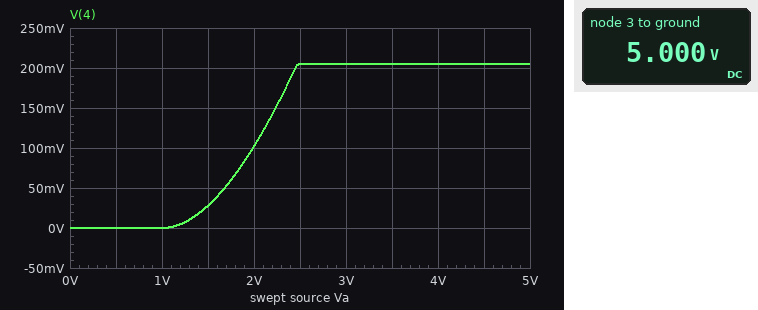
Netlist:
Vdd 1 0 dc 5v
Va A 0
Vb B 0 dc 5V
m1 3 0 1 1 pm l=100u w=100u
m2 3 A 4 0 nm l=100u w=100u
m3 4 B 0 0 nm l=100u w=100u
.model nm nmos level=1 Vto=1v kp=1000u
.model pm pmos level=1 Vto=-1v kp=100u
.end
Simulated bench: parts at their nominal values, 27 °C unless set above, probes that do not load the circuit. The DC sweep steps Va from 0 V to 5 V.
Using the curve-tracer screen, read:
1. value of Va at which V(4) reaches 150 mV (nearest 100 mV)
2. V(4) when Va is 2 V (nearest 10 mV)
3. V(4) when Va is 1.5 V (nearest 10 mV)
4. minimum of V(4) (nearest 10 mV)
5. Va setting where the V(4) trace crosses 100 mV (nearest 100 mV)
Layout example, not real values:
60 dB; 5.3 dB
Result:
2.2 V; 100 mV; 30 mV; 0 V; 2.0 V
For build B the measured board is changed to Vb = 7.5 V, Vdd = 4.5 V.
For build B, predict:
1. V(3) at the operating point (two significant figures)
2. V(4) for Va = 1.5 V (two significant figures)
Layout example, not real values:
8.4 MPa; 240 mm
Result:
4.5 V; 18 mV
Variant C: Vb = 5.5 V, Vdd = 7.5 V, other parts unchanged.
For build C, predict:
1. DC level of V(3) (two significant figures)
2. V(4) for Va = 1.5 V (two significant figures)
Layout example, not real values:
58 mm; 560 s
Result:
7.5 V; 25 mV
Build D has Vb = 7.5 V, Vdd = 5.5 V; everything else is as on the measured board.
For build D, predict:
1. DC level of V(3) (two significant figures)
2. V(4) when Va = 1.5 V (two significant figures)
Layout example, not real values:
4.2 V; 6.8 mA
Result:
5.5 V; 18 mV
